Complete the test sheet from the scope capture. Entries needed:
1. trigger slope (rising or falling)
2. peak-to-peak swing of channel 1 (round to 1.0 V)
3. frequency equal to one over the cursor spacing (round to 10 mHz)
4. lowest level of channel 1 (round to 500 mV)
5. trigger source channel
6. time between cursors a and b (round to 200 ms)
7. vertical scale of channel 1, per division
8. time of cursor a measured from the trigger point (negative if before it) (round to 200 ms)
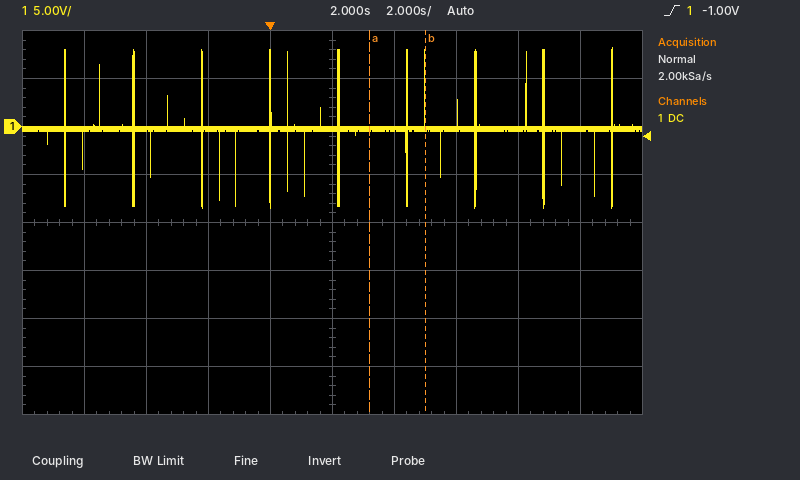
rising
17.0 V
560 mHz
-8.5 V
channel 1
1.8 s
5 V
+3.2 s
